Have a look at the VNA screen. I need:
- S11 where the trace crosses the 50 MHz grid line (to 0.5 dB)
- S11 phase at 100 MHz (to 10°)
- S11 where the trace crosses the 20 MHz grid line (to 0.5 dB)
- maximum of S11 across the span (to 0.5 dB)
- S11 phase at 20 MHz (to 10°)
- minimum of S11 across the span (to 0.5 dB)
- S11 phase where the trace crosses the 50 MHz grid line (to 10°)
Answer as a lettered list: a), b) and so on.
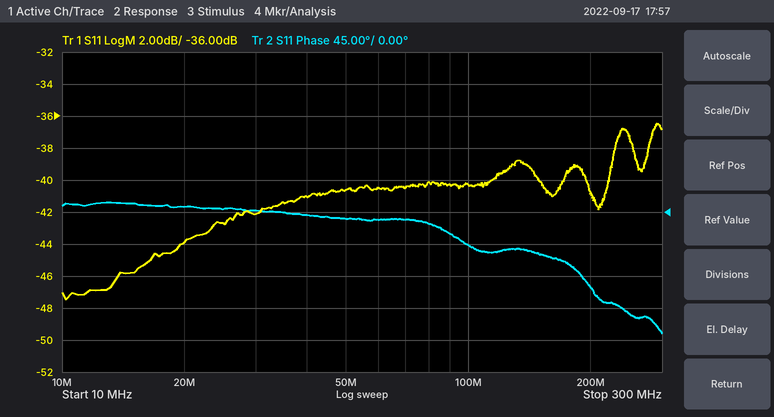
a) -40.5 dB
b) -50°
c) -44.0 dB
d) -36.5 dB
e) 10°
f) -47.5 dB
g) -10°
